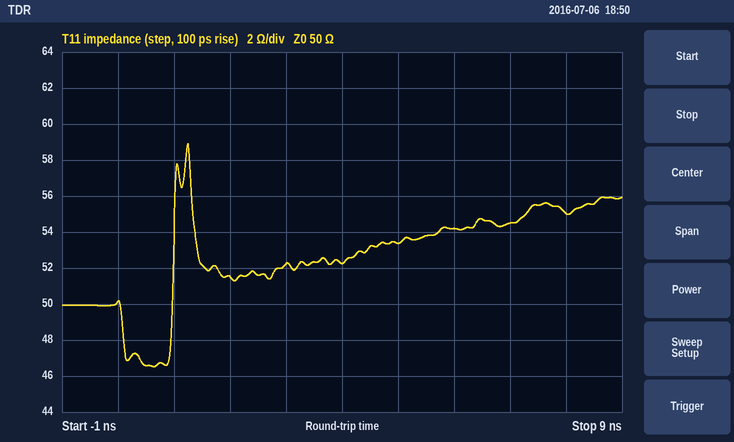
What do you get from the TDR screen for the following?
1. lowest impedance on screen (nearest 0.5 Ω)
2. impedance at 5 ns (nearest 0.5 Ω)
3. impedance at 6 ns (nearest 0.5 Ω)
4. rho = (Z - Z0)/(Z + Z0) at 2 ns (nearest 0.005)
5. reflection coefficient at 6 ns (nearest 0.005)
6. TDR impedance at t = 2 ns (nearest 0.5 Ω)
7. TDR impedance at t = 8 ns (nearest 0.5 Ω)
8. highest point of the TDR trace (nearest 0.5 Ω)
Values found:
46.5 Ω
53.5 Ω
54.0 Ω
+0.015
+0.040
51.5 Ω
55.0 Ω
59.0 Ω
